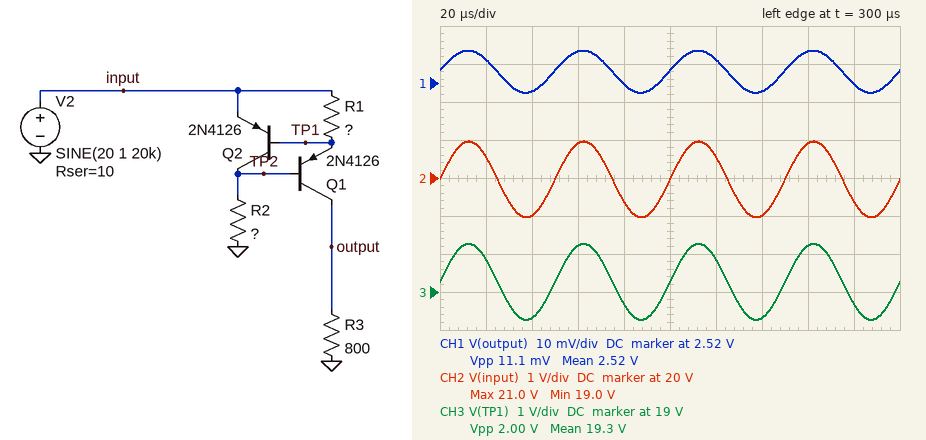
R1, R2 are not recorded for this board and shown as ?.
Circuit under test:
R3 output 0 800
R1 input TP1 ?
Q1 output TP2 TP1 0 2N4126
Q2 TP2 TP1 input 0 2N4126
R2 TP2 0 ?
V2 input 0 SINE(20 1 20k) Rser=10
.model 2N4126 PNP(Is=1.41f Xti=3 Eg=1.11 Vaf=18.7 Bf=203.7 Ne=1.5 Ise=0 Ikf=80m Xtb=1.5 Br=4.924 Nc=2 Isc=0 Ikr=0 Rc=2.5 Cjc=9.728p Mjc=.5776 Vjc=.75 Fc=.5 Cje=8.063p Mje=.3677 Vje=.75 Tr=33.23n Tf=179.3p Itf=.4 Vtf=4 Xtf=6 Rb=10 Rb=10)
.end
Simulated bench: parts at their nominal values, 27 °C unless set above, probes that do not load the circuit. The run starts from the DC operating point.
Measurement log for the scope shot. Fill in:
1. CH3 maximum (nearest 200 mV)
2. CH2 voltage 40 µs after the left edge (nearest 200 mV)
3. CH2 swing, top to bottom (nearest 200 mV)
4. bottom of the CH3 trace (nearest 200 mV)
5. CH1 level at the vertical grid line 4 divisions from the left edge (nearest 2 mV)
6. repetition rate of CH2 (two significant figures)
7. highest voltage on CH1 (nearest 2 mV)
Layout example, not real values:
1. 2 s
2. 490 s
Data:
1. 20.2 V
2. 19.0 V
3. 2.0 V
4. 18.2 V
5. 2.520 V
6. 20 kHz
7. 2.528 V
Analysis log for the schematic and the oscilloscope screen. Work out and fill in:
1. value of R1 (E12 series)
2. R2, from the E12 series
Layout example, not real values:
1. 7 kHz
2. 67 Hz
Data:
1. 220 Ω
2. 27 kΩ
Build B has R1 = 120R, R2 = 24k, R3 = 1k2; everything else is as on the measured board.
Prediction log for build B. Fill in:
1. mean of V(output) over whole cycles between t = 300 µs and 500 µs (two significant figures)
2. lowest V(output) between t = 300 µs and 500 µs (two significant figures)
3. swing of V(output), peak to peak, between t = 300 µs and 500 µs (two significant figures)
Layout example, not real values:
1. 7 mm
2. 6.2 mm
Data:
1. 7.0 V
2. 6.9 V
3. 31 mV
